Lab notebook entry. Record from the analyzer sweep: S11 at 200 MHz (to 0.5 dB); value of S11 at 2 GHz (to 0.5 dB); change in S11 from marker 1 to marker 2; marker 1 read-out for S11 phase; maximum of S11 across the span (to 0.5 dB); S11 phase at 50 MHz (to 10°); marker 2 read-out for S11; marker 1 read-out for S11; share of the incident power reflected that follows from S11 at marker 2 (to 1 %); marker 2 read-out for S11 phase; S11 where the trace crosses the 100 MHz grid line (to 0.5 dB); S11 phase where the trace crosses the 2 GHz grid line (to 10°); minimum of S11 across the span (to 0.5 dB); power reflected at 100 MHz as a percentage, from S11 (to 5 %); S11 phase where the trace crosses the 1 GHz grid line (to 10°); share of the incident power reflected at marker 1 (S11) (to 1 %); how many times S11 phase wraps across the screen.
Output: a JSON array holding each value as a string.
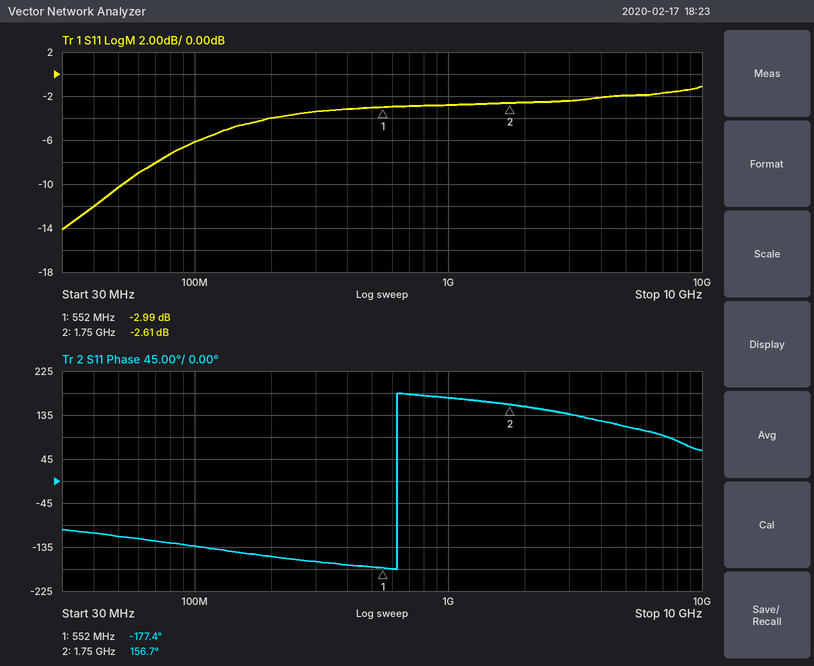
["-4.0 dB", "-2.5 dB", "0.38 dB", "-177.4°", "-1.0 dB", "-110°", "-2.61 dB", "-2.99 dB", "55 %", "156.7°", "-6.0 dB", "150°", "-14.0 dB", "25 %", "170°", "50 %", "1"]
